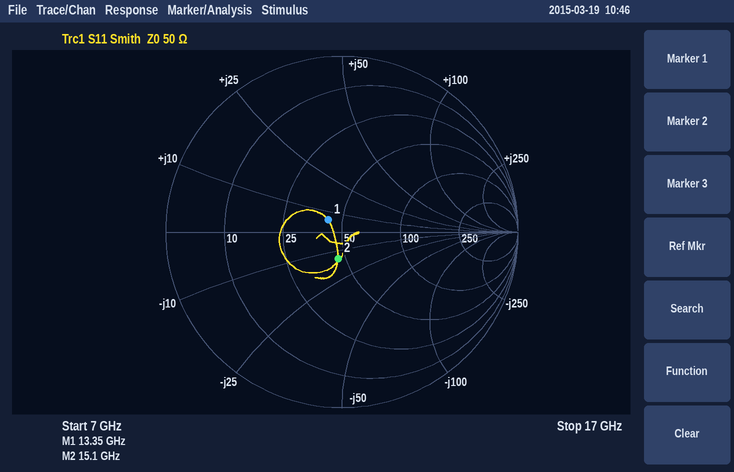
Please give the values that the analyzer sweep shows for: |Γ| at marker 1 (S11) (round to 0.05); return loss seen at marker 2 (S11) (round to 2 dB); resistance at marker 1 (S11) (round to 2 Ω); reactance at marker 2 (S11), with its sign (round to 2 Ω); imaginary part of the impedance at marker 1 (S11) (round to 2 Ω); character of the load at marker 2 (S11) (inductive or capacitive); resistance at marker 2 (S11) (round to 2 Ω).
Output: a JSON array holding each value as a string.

["0.10", "16 dB", "42 Ω", "-14 Ω", "+6 Ω", "capacitive", "46 Ω"]
